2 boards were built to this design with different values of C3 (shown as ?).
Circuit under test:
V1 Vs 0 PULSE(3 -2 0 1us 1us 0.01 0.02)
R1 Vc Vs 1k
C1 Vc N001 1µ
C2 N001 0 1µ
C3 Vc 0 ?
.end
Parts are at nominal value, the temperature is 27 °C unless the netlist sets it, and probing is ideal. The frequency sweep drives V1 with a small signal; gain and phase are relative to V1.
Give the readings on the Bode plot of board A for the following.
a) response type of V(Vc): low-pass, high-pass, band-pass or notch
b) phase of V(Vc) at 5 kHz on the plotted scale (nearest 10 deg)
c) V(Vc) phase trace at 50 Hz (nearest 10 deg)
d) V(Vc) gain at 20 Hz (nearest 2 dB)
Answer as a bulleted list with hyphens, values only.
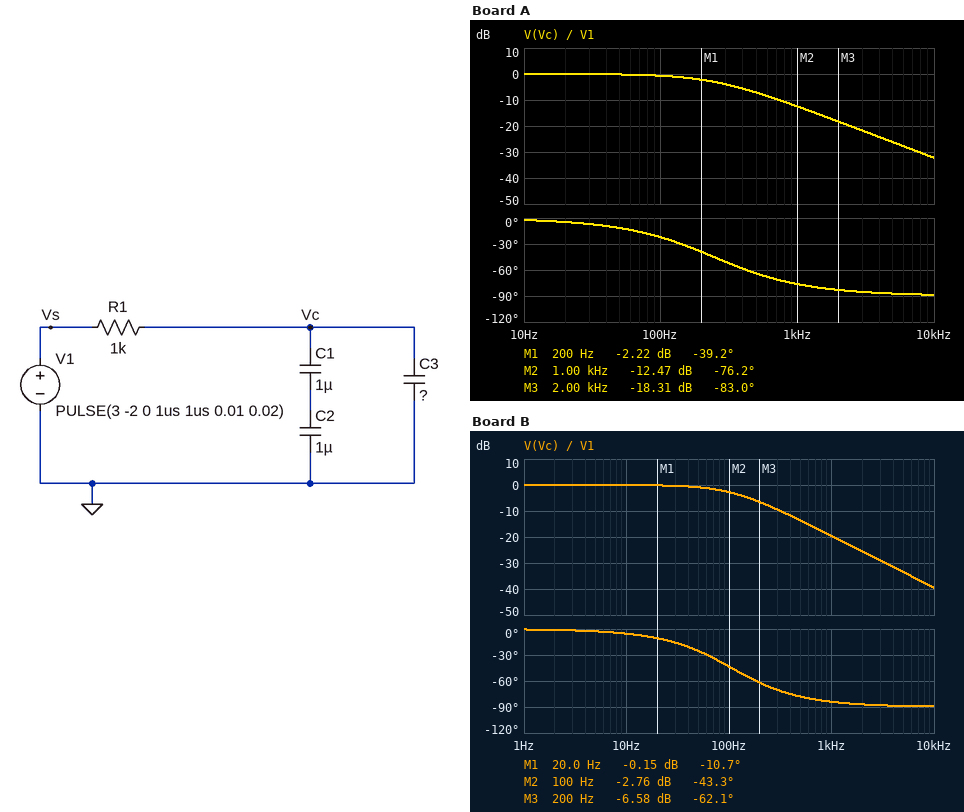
- low-pass
- -90 deg
- -10 deg
- 0 dB
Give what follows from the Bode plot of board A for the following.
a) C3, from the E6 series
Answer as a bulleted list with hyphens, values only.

- 150 nF
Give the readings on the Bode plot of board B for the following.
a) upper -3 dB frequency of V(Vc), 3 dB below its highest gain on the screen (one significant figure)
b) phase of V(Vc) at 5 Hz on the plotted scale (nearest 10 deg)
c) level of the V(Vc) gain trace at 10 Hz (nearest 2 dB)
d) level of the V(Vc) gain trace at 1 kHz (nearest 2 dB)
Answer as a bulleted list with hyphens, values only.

- 100 Hz
- 0 deg
- 0 dB
- -20 dB
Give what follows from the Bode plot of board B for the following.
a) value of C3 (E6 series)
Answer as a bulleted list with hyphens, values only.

- 1 µF
